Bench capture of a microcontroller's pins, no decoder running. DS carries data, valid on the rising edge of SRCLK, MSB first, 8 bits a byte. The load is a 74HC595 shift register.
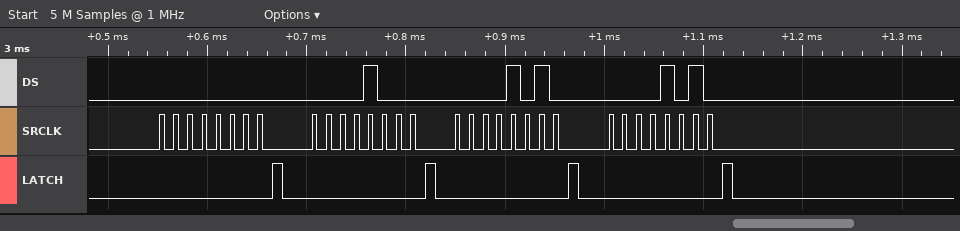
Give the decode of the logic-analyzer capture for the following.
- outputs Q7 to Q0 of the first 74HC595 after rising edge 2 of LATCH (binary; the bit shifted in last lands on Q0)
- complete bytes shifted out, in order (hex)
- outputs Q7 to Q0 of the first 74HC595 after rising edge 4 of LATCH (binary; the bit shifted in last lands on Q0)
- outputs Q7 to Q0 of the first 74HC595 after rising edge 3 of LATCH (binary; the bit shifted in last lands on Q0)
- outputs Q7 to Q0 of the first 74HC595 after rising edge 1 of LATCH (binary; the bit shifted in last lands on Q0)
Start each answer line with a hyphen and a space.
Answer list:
- 00001000
- 00 08 0A 0A
- 00001010
- 00001010
- 00000000
